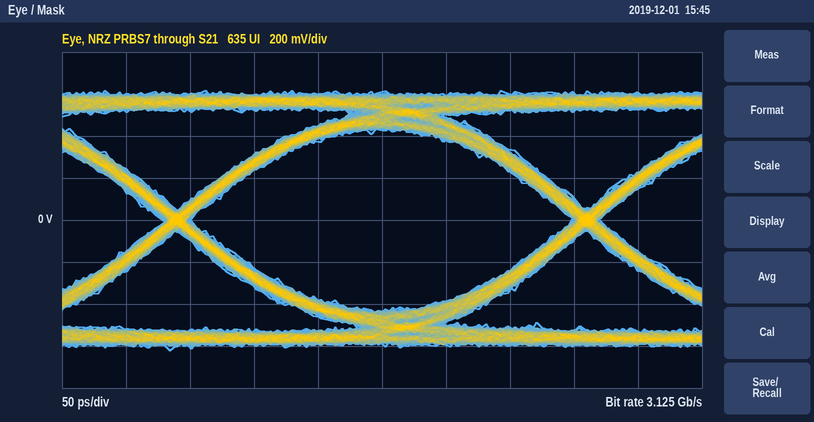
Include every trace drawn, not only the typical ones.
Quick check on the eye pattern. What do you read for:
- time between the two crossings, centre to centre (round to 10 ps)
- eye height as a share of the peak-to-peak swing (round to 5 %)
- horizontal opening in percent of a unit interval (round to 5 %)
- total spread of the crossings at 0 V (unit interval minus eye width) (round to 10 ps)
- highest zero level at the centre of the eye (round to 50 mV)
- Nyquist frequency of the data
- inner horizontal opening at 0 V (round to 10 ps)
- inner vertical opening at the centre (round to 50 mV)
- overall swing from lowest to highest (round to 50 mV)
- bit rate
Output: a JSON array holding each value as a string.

["320 ps", "70 %", "95 %", "20 ps", "-450 mV", "1.5625 GHz", "300 ps", "850 mV", "1.25 V", "3.125 Gb/s"]
